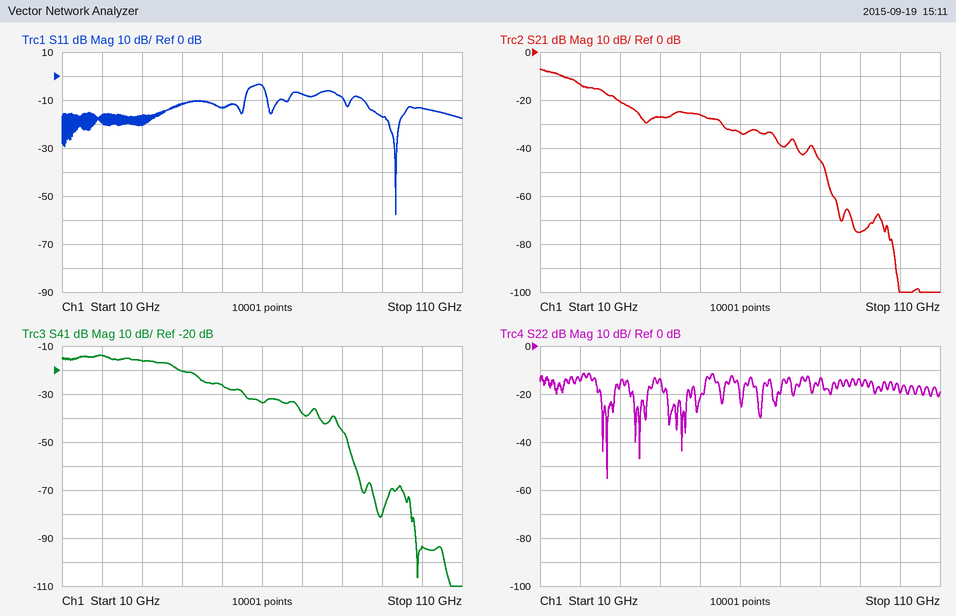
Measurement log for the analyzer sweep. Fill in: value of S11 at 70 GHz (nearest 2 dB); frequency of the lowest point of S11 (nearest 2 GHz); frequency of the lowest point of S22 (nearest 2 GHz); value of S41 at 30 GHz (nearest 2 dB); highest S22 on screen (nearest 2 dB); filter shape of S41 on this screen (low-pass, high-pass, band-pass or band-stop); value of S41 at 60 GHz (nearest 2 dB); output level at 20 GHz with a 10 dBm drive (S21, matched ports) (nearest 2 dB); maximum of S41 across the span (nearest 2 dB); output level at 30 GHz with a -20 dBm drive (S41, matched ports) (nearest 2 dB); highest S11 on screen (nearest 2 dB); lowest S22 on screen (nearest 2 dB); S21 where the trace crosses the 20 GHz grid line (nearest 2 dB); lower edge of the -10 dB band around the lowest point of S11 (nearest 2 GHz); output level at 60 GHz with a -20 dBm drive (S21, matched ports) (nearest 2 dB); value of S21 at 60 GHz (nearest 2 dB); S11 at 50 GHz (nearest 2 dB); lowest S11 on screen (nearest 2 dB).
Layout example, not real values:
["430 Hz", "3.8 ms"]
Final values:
["-8 dB", "94 GHz", "26 GHz", "-16 dB", "-12 dB", "low-pass", "-34 dB", "-4 dBm", "-14 dB", "-36 dBm", "-4 dB", "-56 dB", "-14 dB", "86 GHz", "-54 dBm", "-34 dB", "-14 dB", "-58 dB"]
